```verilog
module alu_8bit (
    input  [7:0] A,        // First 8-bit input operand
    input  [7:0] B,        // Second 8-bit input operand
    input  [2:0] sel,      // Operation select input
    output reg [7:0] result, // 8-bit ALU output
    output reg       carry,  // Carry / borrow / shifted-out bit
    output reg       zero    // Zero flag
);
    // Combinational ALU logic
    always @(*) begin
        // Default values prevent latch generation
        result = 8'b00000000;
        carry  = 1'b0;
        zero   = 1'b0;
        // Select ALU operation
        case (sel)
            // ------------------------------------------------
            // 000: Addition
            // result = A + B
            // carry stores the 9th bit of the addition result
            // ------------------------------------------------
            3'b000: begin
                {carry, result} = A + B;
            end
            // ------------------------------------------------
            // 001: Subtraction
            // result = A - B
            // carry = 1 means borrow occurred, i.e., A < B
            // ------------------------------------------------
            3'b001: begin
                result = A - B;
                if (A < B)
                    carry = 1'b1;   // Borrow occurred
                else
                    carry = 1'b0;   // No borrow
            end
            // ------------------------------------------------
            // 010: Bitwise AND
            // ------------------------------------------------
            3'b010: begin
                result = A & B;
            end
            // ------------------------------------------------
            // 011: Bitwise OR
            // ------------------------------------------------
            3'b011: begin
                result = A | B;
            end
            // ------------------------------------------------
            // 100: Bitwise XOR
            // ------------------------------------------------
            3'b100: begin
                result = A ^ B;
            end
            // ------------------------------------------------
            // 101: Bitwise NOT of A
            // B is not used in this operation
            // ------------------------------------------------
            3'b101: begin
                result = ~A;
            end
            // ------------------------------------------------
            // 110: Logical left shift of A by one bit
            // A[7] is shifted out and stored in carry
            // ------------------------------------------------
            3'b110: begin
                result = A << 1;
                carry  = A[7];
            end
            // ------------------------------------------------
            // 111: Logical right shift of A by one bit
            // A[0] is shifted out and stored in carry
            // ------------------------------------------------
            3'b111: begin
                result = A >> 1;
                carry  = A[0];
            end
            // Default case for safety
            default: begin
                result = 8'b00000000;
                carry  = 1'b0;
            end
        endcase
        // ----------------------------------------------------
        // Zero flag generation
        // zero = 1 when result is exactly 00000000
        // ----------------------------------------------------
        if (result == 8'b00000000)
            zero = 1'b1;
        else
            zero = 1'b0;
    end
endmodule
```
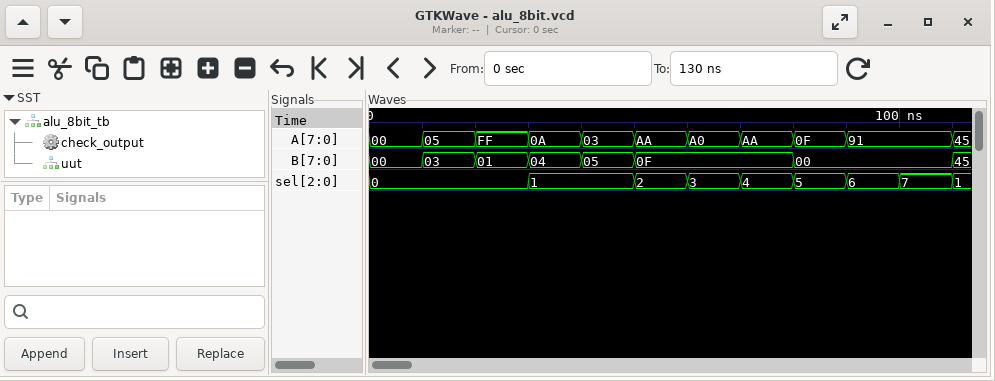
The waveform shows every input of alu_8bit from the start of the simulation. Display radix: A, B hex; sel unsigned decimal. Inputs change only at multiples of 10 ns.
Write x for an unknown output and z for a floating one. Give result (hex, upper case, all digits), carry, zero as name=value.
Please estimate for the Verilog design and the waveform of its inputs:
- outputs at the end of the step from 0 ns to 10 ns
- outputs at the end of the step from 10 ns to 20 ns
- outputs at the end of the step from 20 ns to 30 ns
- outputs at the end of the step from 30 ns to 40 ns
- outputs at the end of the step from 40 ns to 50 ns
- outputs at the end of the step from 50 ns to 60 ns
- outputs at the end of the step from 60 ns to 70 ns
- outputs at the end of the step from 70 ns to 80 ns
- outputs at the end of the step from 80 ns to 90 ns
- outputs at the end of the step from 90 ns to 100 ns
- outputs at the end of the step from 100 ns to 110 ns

result=00, carry=0, zero=1
result=08, carry=0, zero=0
result=00, carry=1, zero=1
result=06, carry=0, zero=0
result=FE, carry=1, zero=0
result=0A, carry=0, zero=0
result=AF, carry=0, zero=0
result=A5, carry=0, zero=0
result=F0, carry=0, zero=0
result=22, carry=1, zero=0
result=48, carry=1, zero=0
